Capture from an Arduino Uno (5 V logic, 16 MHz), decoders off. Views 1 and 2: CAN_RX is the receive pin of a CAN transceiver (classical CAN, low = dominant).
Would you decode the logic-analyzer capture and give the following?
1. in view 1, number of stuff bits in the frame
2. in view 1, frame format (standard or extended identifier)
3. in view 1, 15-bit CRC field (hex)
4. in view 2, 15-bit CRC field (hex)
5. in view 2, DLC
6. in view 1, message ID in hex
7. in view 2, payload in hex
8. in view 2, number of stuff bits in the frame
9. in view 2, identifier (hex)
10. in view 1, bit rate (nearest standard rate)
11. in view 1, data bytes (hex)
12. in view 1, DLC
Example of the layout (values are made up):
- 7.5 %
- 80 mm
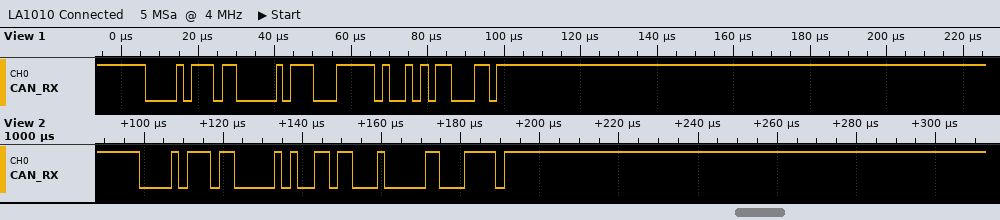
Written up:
- 2
- standard
- 0x72B1
- 0x1047
- 1
- 0x0BB
- 36
- 2
- 0x0BB
- 500 kbit/s
- C7
- 1
